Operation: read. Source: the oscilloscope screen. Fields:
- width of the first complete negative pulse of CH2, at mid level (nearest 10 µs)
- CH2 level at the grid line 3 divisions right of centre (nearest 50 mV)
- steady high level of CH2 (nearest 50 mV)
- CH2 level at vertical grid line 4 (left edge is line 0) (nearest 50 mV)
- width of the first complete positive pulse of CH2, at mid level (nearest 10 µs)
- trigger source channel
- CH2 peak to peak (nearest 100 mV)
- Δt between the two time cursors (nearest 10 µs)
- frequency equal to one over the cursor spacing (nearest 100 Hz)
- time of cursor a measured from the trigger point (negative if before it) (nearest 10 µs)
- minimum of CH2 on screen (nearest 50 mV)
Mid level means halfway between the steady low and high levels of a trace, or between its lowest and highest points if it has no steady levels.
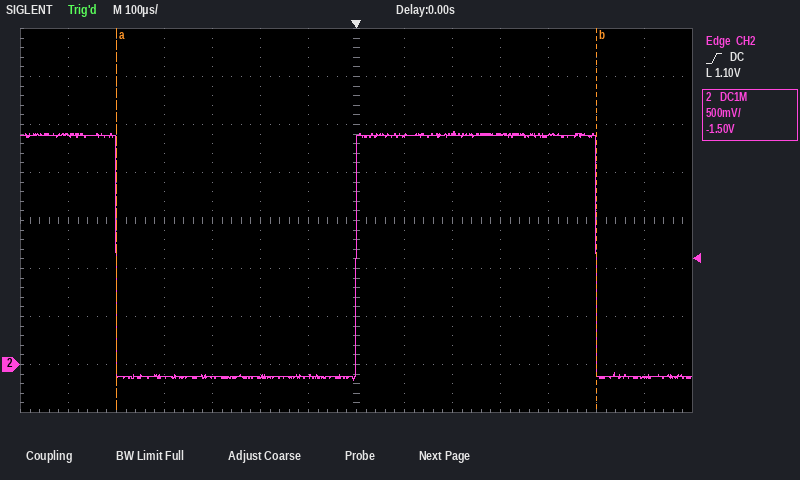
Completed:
500 µs
2.40 V
2.40 V
-150 mV
500 µs
CH2
2.60 V
1.00 ms
1.0 kHz
-500 µs
-150 mV
